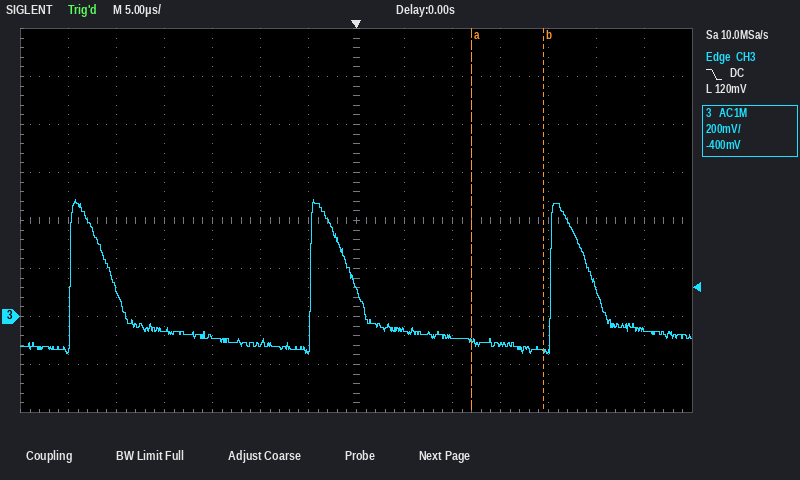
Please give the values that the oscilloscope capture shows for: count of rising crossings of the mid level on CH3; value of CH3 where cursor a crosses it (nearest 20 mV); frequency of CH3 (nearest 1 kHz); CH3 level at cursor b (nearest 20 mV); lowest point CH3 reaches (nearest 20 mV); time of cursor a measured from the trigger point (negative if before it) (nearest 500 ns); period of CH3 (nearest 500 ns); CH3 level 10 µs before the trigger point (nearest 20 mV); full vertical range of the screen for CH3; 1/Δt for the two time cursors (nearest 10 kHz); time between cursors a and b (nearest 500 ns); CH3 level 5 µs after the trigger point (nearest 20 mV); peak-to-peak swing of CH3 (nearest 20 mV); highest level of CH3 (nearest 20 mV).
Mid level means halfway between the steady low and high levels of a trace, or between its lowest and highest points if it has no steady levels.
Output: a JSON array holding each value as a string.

["3", "-100 mV", "40 kHz", "-140 mV", "-160 mV", "+12.0 µs", "25.0 µs", "-120 mV", "1.6 V", "130 kHz", "7.5 µs", "-60 mV", "640 mV", "480 mV"]
